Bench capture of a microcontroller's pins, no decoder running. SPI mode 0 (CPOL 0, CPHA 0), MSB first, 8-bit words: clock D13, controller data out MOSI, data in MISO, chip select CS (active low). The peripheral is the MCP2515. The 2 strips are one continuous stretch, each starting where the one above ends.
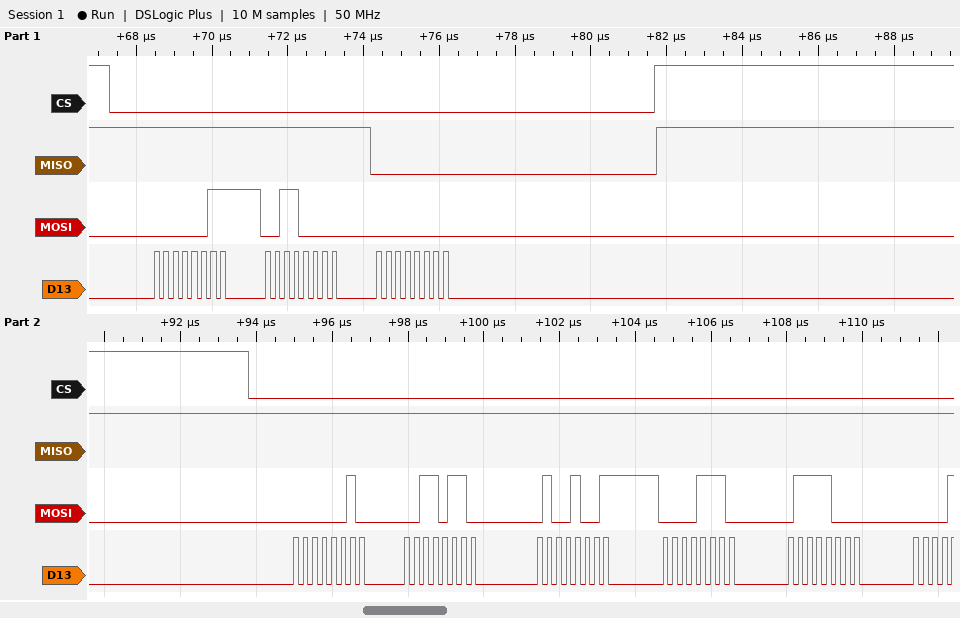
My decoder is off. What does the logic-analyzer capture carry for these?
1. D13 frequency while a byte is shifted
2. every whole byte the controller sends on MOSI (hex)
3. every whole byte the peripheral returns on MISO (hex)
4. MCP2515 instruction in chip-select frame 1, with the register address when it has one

4 MHz
03 30 00 02 36 49 0E 78
FF FF 00 FF FF FF FF FF
READ 0x30
